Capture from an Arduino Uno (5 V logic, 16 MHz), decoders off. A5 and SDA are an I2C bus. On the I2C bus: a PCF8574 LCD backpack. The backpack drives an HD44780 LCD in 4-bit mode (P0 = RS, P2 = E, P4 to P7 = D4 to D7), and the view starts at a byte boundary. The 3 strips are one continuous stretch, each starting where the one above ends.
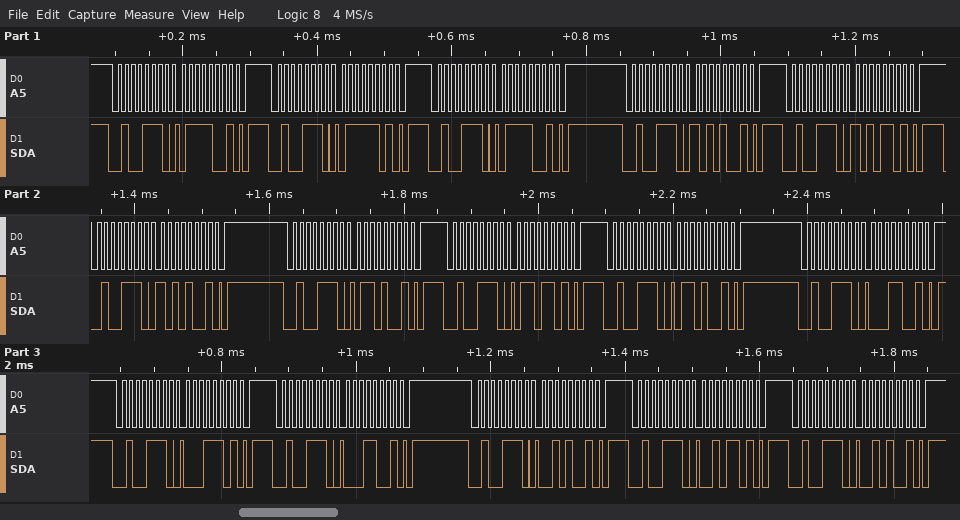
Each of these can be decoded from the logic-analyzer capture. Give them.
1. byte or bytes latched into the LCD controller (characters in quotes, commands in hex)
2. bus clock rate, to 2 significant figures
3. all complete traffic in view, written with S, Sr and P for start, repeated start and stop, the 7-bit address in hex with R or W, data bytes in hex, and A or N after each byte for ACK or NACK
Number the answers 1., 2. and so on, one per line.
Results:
1. 'z' 'a'
2. 100 kHz
3. S 27W A 79 A P S 27W A 7D A P S 27W A 79 A P S 27W A A9 A P S 27W A AD A P S 27W A A9 A P S 27W A 69 A P S 27W A 6D A P S 27W A 69 A P S 27W A 19 A P S 27W A 1D A P S 27W A 19 A P S 27W A 29 A P S 27W A 2D A P S 27W A 29 A P
